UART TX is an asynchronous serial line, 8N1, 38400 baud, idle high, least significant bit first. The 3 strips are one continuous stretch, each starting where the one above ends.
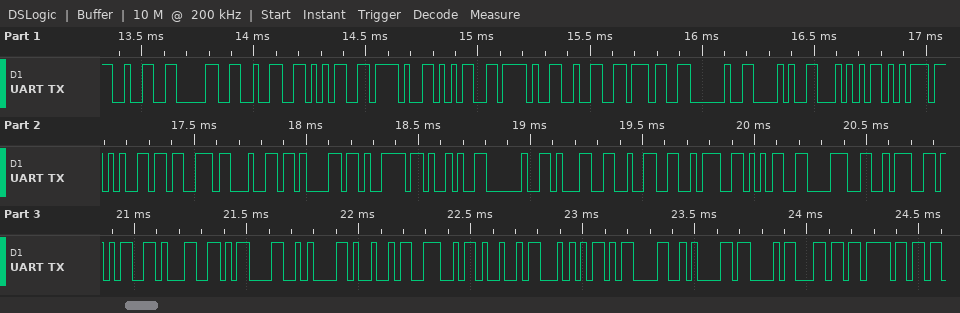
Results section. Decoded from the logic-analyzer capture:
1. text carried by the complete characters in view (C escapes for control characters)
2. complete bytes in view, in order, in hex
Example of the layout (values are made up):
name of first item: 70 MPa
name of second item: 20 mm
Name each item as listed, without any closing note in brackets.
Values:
text carried by the complete characters in view: "2025/5/27 (Tuesday) 12:58:51\r\nINIT\r\nClo"
complete bytes in view, in order, in hex: 0x32 0x30 0x32 0x35 0x2F 0x35 0x2F 0x32 0x37 0x20 0x28 0x54 0x75 0x65 0x73 0x64 0x61 0x79 0x29 0x20 0x31 0x32 0x3A 0x35 0x38 0x3A 0x35 0x31 0x0D 0x0A 0x49 0x4E 0x49 0x54 0x0D 0x0A 0x43 0x6C 0x6F
